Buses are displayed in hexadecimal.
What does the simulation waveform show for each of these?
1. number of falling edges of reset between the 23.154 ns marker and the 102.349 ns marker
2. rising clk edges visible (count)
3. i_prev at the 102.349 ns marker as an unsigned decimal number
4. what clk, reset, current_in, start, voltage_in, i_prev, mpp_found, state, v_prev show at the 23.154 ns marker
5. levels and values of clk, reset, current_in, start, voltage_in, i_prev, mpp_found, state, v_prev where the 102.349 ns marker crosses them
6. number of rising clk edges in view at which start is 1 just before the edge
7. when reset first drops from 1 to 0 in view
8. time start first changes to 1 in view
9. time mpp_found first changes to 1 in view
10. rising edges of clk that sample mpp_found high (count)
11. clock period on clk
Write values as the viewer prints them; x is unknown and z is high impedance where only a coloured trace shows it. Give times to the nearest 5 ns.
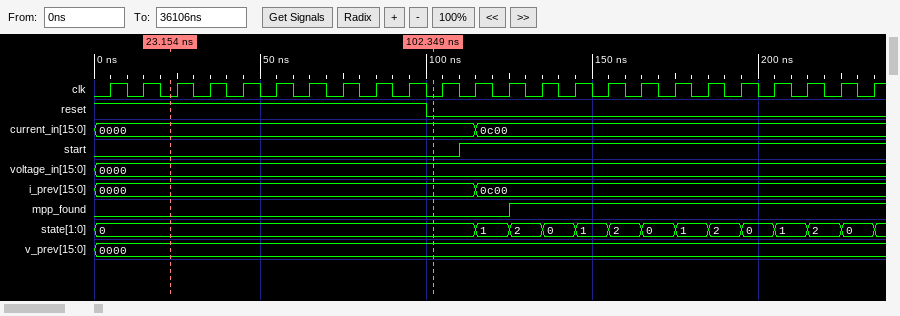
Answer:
1
24
0
clk=0, reset=1, current_in=0000, start=0, voltage_in=0000, i_prev=0000, mpp_found=0, state=0, v_prev=0000
clk=0, reset=0, current_in=0000, start=0, voltage_in=0000, i_prev=0000, mpp_found=0, state=0, v_prev=0000
13
100 ns
110 ns
125 ns
11
10 ns
